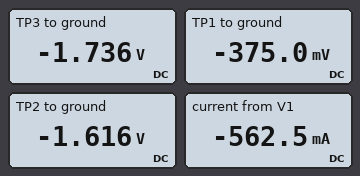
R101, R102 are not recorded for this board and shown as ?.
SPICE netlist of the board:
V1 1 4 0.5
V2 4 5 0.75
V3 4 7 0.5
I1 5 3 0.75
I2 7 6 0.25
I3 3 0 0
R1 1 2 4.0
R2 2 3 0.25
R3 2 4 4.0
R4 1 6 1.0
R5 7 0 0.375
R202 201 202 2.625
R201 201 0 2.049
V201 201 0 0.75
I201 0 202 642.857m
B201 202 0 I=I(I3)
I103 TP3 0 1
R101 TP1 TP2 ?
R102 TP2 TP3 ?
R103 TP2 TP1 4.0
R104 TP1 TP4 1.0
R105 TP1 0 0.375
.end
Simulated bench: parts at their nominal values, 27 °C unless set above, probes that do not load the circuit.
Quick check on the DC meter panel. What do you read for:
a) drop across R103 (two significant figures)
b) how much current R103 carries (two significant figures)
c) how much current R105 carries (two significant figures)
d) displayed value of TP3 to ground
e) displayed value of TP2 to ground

1.2 V
310 mA
1.0 A
-1.736 V
-1.616 V
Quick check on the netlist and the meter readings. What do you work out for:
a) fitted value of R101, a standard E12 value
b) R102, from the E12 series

1.8 Ω
0.12 Ω
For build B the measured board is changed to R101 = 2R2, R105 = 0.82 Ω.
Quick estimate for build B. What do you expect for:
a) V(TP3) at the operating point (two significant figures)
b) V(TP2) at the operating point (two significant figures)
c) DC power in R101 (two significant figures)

-2.4 V
-2.2 V
920 mW
